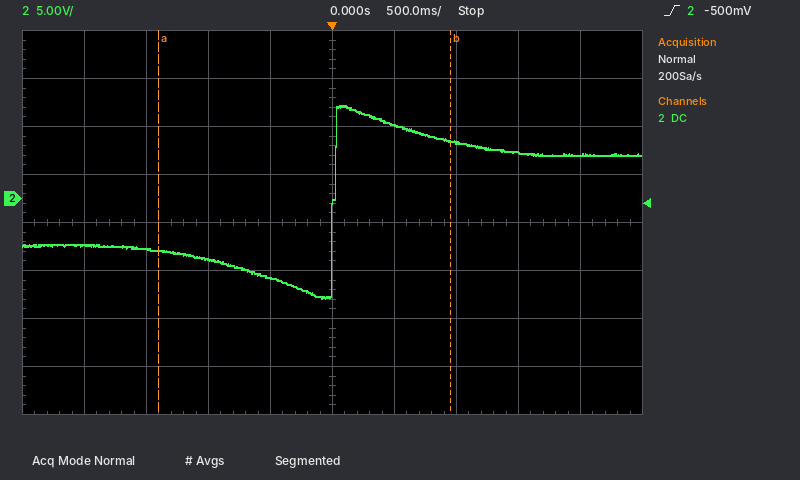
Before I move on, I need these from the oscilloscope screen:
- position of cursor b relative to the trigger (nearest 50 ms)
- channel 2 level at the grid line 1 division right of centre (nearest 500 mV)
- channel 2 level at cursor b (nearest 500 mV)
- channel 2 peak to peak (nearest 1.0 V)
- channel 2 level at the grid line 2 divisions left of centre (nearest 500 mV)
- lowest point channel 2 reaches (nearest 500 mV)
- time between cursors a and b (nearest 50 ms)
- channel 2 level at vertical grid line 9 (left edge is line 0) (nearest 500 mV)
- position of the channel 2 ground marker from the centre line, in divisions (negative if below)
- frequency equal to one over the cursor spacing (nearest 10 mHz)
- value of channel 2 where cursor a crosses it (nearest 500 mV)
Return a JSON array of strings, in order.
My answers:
["+950 ms", "7.5 V", "6.0 V", "20.0 V", "-6.5 V", "-10.5 V", "2.35 s", "4.5 V", "+0.5 div", "430 mHz", "-5.5 V"]
